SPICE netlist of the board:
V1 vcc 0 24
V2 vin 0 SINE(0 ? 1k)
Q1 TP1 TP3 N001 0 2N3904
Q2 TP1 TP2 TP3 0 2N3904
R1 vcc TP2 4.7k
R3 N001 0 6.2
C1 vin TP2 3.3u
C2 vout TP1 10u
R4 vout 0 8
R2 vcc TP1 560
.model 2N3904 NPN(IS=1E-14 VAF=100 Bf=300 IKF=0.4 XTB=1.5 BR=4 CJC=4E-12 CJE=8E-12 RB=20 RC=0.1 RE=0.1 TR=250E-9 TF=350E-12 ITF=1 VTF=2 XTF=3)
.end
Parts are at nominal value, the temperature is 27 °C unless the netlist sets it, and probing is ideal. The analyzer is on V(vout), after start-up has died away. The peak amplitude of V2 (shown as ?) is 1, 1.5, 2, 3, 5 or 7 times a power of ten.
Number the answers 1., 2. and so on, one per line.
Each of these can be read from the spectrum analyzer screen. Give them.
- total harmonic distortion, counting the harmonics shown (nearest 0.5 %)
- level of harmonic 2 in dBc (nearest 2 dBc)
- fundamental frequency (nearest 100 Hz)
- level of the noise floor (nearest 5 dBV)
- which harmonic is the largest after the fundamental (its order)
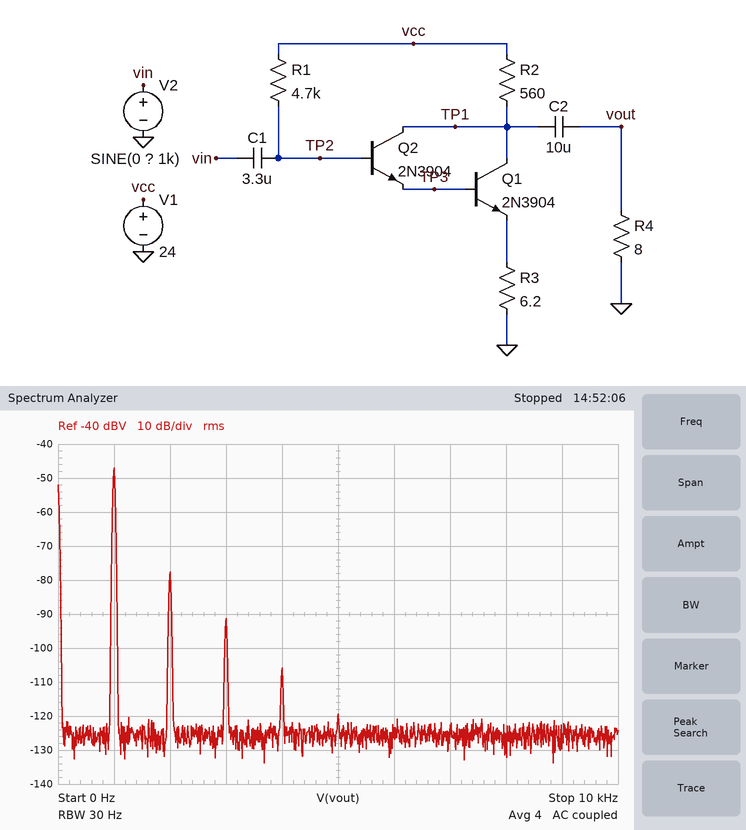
1. 3.0 %
2. -30 dBc
3. 1.0 kHz
4. -125 dBV
5. 2
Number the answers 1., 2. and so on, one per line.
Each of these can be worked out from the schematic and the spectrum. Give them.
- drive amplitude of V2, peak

1. 150 mV
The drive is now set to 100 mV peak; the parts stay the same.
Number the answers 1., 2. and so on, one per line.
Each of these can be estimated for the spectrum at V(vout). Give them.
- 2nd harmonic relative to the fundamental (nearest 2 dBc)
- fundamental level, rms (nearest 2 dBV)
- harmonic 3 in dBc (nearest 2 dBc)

1. -34 dBc
2. -50 dBV
3. -52 dBc
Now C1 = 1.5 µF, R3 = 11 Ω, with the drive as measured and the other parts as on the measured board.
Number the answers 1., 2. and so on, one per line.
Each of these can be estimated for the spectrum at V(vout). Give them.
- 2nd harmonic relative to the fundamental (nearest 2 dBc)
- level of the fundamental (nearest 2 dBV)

1. -42 dBc
2. -50 dBV
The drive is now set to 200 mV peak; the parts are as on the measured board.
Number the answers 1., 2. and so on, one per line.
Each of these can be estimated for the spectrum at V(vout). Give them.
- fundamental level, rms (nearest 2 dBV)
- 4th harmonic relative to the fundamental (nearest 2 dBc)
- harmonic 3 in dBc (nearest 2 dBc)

1. -44 dBV
2. -50 dBc
3. -38 dBc
